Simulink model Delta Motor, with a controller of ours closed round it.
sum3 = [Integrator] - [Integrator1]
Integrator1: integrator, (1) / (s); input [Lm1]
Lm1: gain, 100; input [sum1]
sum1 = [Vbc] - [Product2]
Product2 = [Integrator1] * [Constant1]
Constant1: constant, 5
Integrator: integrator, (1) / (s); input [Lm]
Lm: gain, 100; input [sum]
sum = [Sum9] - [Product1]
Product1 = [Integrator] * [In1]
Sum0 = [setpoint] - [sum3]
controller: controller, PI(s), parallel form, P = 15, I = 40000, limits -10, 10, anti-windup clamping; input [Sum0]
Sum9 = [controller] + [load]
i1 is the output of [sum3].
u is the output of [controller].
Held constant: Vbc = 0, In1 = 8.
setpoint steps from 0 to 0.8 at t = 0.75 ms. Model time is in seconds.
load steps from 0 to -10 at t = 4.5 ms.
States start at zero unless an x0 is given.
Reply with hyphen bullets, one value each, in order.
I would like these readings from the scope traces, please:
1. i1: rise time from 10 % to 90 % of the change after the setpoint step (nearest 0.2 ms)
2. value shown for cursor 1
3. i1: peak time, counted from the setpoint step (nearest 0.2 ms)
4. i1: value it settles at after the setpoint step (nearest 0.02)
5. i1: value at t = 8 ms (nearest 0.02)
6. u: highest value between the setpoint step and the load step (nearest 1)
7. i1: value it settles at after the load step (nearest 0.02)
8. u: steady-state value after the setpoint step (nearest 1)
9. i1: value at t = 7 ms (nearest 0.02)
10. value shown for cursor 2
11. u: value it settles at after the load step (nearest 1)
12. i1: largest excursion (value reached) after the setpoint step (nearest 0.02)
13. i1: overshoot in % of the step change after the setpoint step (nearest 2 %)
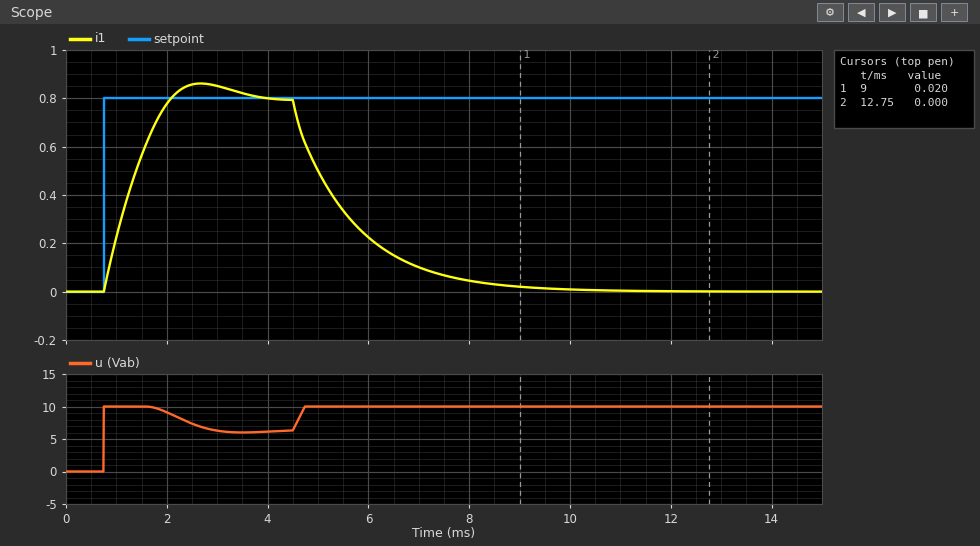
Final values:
- 1.0 ms
- 0.020
- 2.0 ms
- 0.80
- 0.04
- 10
- 0.00
- 6
- 0.10
- 0.000
- 10
- 0.86
- 8 %
